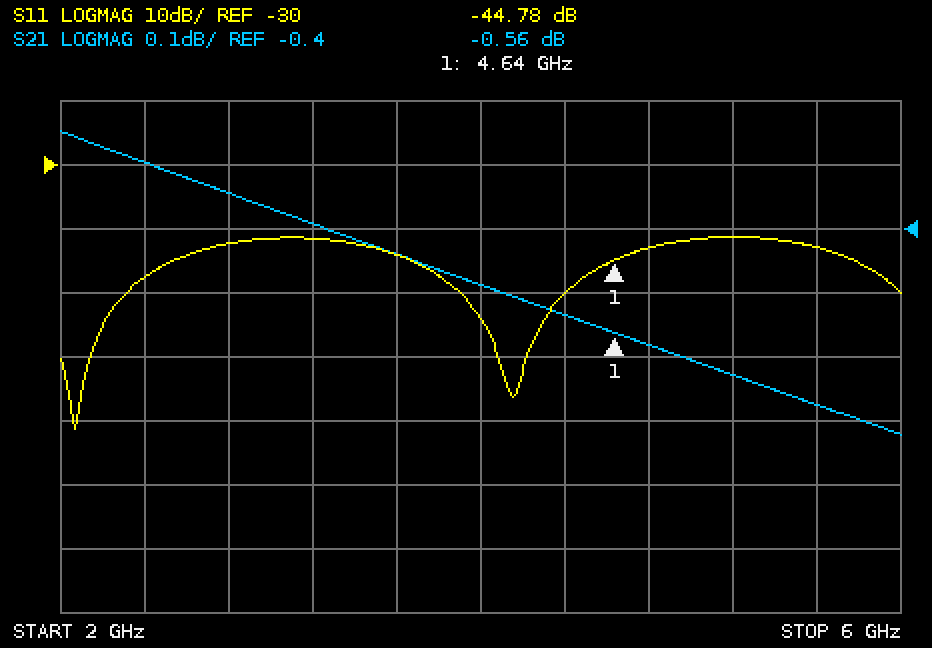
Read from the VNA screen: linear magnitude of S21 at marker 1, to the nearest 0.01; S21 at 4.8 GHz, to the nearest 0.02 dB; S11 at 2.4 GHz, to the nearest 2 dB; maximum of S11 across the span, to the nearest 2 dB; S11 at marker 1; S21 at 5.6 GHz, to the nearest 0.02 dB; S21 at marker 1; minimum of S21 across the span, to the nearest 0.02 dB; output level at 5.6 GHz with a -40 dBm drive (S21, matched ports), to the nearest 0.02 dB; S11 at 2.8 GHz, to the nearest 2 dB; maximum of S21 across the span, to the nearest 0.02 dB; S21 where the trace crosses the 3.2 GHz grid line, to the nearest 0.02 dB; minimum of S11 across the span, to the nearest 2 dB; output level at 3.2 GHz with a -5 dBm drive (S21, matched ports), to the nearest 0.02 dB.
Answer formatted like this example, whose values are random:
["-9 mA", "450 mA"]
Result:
["0.94", "-0.58 dB", "-48 dB", "-42 dB", "-44.78 dB", "-0.68 dB", "-0.56 dB", "-0.72 dB", "-40.68 dBm", "-42 dB", "-0.24 dB", "-0.40 dB", "-72 dB", "-5.40 dBm"]
